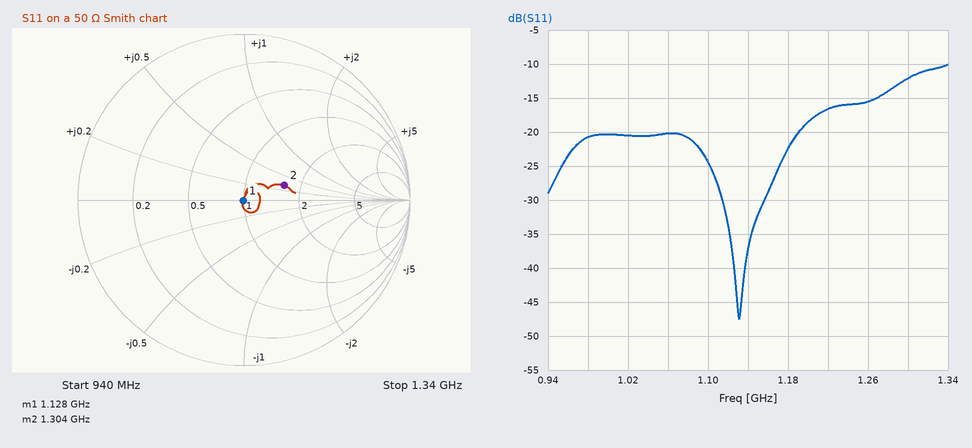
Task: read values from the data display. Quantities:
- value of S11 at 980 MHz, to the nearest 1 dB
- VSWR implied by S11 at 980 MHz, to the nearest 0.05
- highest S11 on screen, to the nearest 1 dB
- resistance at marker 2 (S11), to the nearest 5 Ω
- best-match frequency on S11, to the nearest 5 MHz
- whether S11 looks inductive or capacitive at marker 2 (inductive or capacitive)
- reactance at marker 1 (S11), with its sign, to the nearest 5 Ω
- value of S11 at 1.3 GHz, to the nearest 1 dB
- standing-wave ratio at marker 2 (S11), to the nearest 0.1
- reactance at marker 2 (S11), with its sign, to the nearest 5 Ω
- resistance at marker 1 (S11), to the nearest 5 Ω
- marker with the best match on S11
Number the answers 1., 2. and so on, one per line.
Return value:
1. -21 dB
2. 1.20
3. -10 dB
4. 80 Ω
5. 1.130 GHz
6. inductive
7. 0 Ω
8. -12 dB
9. 1.7
10. +15 Ω
11. 50 Ω
12. marker 1
